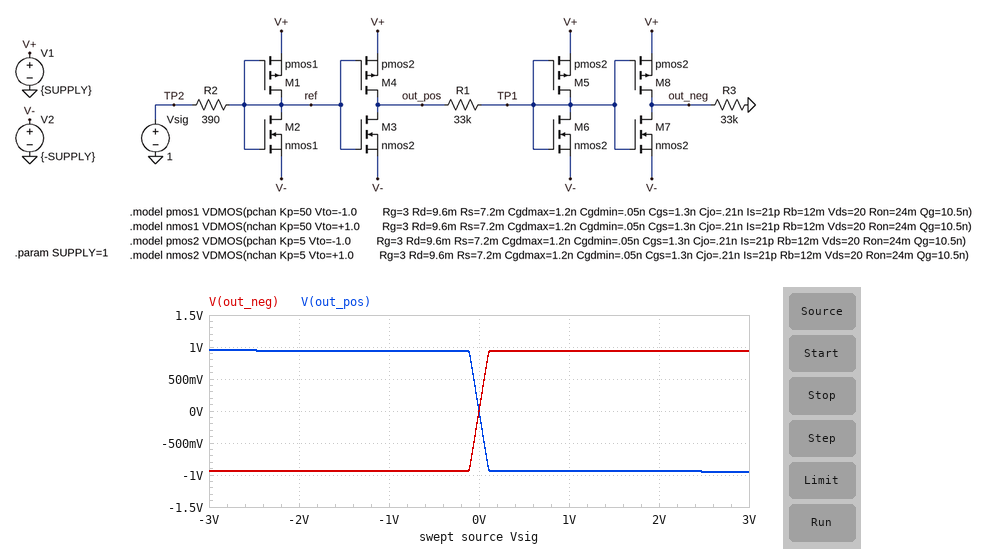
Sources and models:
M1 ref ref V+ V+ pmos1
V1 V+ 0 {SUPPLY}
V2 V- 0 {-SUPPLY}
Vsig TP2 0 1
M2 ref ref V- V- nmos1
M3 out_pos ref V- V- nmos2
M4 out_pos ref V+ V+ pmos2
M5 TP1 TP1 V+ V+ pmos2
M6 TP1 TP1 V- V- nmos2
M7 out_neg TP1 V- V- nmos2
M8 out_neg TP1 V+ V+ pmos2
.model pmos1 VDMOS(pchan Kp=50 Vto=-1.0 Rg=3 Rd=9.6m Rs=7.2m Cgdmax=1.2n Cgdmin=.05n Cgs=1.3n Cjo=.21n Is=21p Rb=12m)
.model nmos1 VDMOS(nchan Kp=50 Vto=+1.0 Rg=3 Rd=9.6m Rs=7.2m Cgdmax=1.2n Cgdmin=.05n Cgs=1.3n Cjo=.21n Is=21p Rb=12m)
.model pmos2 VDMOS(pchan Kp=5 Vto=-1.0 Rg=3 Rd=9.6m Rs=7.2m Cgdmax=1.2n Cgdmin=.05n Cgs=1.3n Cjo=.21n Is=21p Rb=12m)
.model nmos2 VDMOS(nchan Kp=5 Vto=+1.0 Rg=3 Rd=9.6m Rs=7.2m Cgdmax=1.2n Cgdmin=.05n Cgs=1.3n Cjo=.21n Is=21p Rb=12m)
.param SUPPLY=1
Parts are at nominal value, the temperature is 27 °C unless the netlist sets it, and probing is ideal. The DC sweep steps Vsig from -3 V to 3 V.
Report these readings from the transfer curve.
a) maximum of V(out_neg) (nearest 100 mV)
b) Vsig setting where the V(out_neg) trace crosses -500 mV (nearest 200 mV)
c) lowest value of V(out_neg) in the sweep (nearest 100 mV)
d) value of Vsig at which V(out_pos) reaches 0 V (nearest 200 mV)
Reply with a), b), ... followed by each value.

a) 900 mV
b) 0 V
c) -900 mV
d) 0 V
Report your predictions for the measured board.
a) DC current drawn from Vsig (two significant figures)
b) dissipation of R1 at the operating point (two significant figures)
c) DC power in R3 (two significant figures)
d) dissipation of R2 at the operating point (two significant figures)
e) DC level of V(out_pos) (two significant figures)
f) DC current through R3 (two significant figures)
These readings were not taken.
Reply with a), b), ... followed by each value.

a) 2.6 mA
b) 27 µW
c) 26 µW
d) 2.6 mW
e) -940 mV
f) 28 µA
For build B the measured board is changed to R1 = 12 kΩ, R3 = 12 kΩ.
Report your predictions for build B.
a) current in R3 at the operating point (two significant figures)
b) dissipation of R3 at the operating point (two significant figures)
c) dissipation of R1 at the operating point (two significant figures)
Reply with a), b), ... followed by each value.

a) 78 µA
b) 72 µW
c) 73 µW
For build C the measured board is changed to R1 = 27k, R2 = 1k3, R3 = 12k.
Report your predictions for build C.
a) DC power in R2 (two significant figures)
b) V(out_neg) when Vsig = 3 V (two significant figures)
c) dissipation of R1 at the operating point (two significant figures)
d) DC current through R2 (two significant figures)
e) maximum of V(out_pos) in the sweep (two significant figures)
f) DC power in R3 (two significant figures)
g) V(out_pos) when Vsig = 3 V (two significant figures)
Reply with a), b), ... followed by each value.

a) 770 µW
b) 420 mV
c) 32 µW
d) 770 µA
e) 940 mV
f) 14 µW
g) -940 mV
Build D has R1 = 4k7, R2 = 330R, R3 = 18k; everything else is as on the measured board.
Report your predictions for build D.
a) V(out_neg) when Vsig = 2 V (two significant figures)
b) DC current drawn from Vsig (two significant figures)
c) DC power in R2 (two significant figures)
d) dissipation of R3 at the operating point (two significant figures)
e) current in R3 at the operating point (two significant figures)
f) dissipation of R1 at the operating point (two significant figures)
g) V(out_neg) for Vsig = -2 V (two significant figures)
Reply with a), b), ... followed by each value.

a) 940 mV
b) 3.0 mA
c) 3.0 mW
d) 49 µW
e) 52 µA
f) 190 µW
g) -940 mV
